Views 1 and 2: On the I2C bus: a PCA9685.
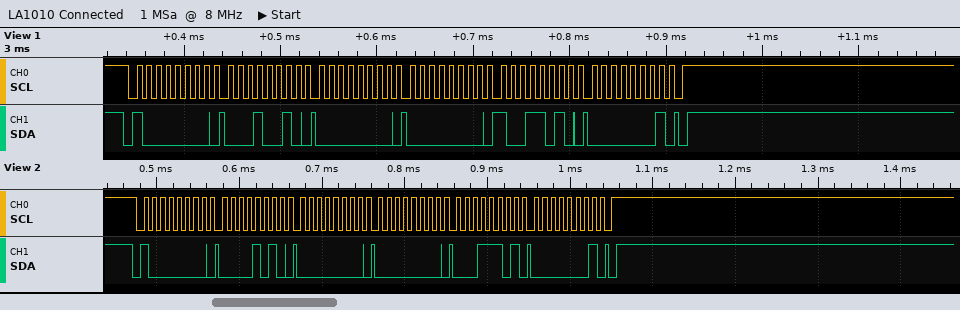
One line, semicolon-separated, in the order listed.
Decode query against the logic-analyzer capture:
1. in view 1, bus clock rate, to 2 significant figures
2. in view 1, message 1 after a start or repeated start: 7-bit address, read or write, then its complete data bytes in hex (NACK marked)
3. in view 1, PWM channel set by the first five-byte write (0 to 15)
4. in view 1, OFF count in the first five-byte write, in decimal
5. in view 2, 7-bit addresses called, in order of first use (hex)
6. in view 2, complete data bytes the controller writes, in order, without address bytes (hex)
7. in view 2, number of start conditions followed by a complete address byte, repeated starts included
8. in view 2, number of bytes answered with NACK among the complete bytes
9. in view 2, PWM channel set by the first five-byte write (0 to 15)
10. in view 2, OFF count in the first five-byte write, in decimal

100 kHz; 0x40 write: 12 00 00 9A 01; 3; 410; 0x40; 0A 00 00 1D 01; 1; 0; 1; 285
